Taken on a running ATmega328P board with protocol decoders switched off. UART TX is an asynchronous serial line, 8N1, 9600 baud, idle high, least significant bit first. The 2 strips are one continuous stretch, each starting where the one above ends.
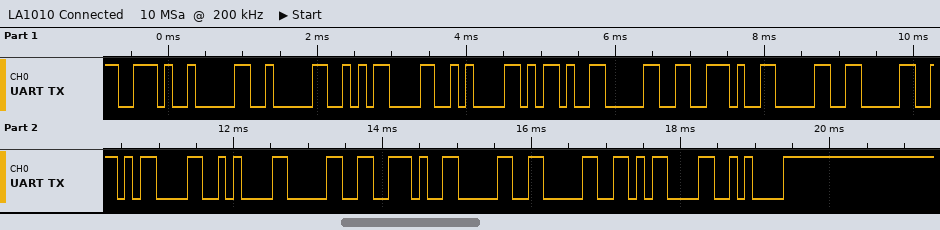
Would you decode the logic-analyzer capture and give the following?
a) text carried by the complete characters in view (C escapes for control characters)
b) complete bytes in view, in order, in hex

".00\r\n-0.00\r\n0.00\r\n"
0x2E 0x30 0x30 0x0D 0x0A 0x2D 0x30 0x2E 0x30 0x30 0x0D 0x0A 0x30 0x2E 0x30 0x30 0x0D 0x0A
